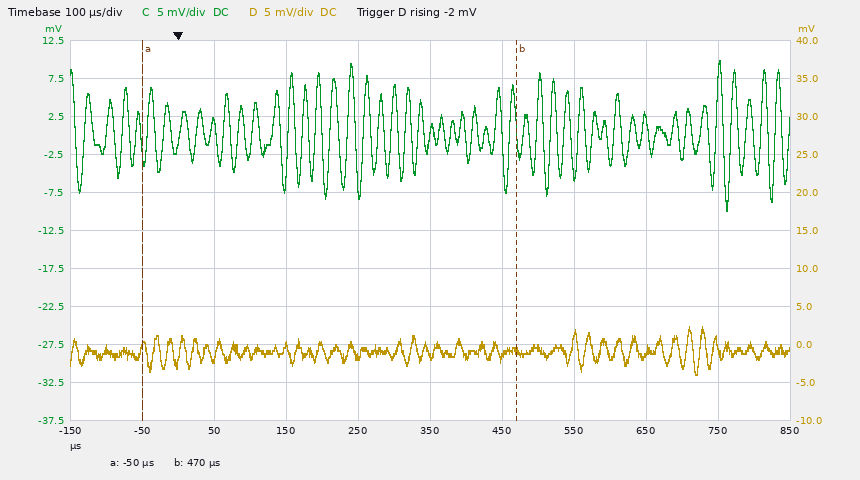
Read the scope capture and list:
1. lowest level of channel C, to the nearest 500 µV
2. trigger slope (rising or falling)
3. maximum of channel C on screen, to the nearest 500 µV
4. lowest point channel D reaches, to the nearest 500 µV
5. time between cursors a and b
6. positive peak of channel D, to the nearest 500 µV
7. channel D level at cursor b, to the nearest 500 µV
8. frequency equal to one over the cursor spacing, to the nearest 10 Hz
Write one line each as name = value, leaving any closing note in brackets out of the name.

lowest level of channel C, to the nearest 500 µV = -10.0 mV
trigger slope = rising
maximum of channel C on screen, to the nearest 500 µV = 10.0 mV
lowest point channel D reaches, to the nearest 500 µV = -4.0 mV
time between cursors a and b = 520 µs
positive peak of channel D, to the nearest 500 µV = 2.5 mV
channel D level at cursor b, to the nearest 500 µV = -1.0 mV
frequency equal to one over the cursor spacing, to the nearest 10 Hz = 1.92 kHz
